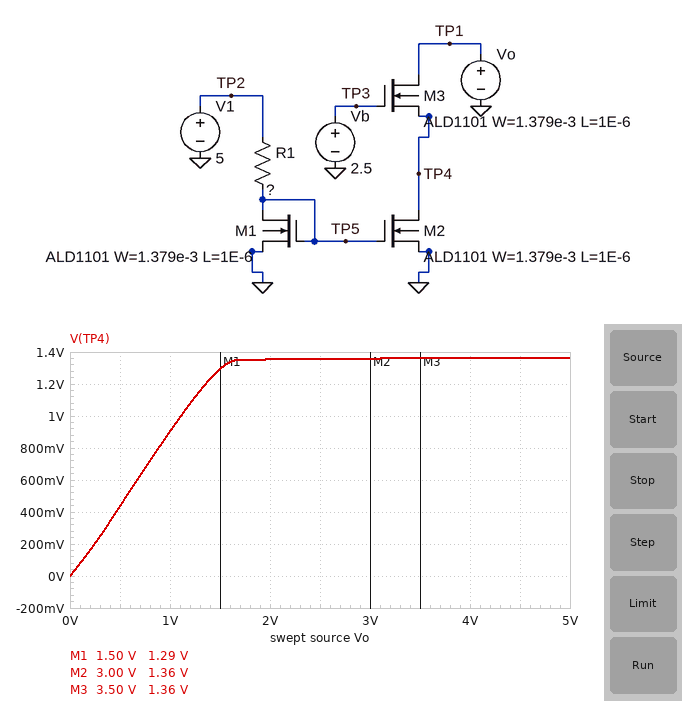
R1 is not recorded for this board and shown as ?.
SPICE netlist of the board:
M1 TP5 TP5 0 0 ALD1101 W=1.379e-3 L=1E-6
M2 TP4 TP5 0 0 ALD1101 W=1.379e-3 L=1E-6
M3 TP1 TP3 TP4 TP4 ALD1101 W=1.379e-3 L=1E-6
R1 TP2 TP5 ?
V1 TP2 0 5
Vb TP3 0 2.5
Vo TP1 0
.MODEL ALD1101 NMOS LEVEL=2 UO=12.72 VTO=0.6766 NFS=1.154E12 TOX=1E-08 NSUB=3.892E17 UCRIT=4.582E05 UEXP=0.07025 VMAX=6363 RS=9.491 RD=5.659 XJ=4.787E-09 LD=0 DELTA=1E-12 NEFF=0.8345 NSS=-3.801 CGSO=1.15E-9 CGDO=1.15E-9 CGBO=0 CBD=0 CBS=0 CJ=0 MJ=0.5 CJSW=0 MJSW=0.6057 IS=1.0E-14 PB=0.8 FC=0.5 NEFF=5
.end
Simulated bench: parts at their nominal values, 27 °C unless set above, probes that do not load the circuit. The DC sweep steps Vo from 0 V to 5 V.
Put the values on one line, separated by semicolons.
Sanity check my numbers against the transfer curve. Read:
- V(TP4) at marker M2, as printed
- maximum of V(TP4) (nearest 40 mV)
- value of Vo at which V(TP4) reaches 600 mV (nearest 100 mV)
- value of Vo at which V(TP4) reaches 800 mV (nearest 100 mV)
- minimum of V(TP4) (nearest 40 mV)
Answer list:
1.36 V; 1.36 V; 700 mV; 900 mV; 0 V
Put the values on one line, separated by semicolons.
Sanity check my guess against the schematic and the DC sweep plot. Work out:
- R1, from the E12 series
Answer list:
8.2 kΩ
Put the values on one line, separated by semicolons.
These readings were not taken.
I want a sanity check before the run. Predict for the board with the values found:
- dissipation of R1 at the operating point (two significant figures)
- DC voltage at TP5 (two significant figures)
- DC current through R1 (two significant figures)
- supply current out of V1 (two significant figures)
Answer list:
1.8 mW; 1.1 V; 470 µA; 470 µA
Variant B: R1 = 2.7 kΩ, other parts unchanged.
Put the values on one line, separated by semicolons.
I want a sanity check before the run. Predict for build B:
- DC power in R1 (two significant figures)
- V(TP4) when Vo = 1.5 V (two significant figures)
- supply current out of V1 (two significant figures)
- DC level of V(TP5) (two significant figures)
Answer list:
4.6 mW; 1.0 V; 1.3 mA; 1.5 V
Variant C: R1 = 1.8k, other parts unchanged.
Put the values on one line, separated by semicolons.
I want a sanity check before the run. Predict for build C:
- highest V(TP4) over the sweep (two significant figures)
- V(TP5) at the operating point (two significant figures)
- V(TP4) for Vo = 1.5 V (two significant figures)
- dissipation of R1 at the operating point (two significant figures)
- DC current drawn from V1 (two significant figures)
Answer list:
890 mV; 1.6 V; 860 mV; 6.3 mW; 1.9 mA
